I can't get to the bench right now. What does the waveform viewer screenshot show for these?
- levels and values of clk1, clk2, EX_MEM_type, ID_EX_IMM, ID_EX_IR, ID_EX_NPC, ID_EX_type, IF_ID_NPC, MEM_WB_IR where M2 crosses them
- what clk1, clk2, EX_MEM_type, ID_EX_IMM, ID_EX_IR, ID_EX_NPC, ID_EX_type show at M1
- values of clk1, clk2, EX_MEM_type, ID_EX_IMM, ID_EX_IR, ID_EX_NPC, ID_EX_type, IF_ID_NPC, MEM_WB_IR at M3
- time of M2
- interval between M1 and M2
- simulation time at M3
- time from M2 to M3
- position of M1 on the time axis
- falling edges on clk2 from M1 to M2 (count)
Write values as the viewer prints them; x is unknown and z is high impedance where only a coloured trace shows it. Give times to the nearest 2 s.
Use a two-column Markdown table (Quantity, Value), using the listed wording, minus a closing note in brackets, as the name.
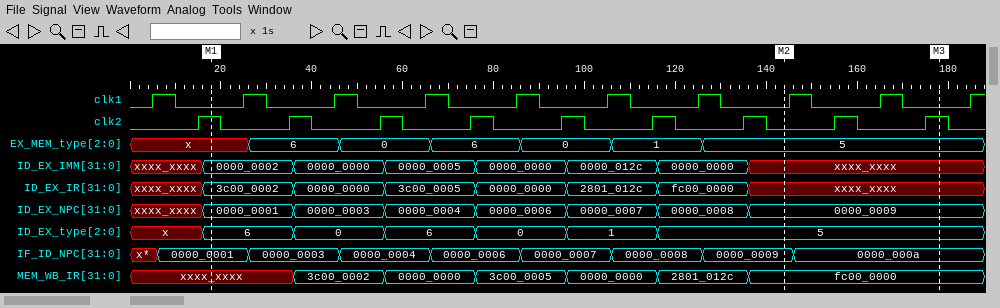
| Quantity | Value |
|---|---|
| levels and values of clk1, clk2, EX_MEM_type, ID_EX_IMM, ID_EX_IR, ID_EX_NPC, ID_EX_type, IF_ID_NPC, MEM_WB_IR where M2 crosses them | clk1=0, clk2=0, EX_MEM_type=5, ID_EX_IMM=xxxx_xxxx, ID_EX_IR=xxxx_xxxx, ID_EX_NPC=0000_0009, ID_EX_type=5, IF_ID_NPC=0000_0009, MEM_WB_IR=fc00_0000 |
| what clk1, clk2, EX_MEM_type, ID_EX_IMM, ID_EX_IR, ID_EX_NPC, ID_EX_type show at M1 | clk1=0, clk2=1, EX_MEM_type=x, ID_EX_IMM=0000_0002, ID_EX_IR=3c00_0002, ID_EX_NPC=0000_0001, ID_EX_type=6 |
| values of clk1, clk2, EX_MEM_type, ID_EX_IMM, ID_EX_IR, ID_EX_NPC, ID_EX_type, IF_ID_NPC, MEM_WB_IR at M3 | clk1=0, clk2=1, EX_MEM_type=5, ID_EX_IMM=xxxx_xxxx, ID_EX_IR=xxxx_xxxx, ID_EX_NPC=0000_0009, ID_EX_type=5, IF_ID_NPC=0000_000a, MEM_WB_IR=fc00_0000 |
| time of M2 | 144 s |
| interval between M1 and M2 | 126 s |
| simulation time at M3 | 178 s |
| time from M2 to M3 | 34 s |
| position of M1 on the time axis | 18 s |
| falling edges on clk2 from M1 to M2 | 7 |
